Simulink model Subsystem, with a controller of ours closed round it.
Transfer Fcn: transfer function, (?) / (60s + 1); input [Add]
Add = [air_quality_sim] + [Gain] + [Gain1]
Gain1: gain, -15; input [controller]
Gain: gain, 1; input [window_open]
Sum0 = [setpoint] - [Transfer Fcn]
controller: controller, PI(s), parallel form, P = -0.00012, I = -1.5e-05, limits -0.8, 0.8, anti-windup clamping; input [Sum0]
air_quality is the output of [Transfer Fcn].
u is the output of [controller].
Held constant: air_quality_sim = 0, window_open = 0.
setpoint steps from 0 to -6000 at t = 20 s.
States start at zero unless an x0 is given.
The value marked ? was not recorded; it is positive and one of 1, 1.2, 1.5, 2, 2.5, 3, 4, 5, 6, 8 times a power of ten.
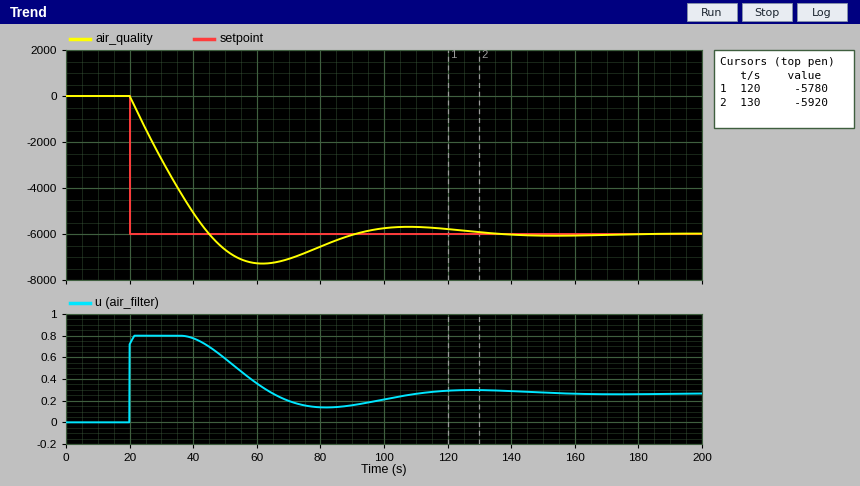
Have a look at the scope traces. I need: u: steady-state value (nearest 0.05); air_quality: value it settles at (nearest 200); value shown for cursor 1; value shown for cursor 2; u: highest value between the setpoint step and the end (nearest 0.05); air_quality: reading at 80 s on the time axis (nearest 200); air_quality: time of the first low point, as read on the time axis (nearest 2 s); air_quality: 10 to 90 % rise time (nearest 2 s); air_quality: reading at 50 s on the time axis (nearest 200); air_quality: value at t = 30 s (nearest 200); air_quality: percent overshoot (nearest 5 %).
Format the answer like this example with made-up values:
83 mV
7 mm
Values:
0.25
-6000
-5780
-5920
0.80
-6600
62 s
20 s
-6600
-2800
20 %
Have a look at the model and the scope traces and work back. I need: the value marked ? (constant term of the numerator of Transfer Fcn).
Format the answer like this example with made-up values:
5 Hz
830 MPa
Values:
1500
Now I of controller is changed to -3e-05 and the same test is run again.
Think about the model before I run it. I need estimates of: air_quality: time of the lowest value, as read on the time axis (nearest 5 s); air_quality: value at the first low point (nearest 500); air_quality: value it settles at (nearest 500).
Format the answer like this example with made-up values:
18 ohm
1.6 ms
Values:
55 s
-7000
-6000
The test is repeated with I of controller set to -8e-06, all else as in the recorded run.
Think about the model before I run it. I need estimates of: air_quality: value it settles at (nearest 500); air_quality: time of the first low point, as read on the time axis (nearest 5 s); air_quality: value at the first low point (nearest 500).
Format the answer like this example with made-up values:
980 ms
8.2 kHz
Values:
-6000
70 s
-7000
